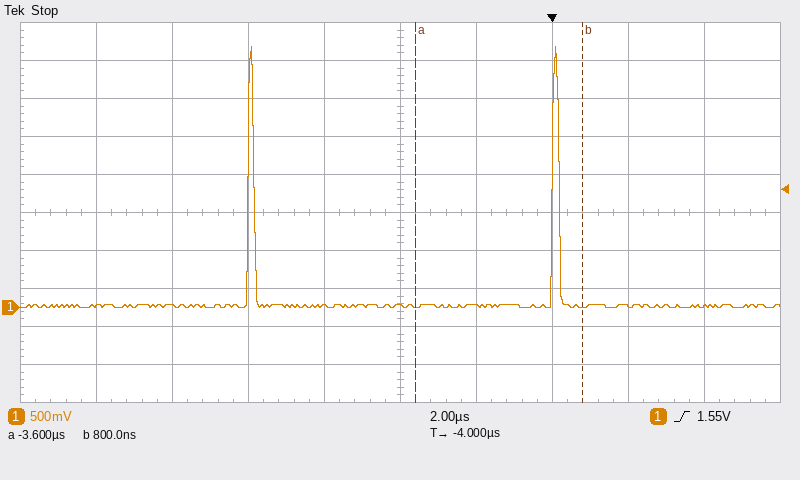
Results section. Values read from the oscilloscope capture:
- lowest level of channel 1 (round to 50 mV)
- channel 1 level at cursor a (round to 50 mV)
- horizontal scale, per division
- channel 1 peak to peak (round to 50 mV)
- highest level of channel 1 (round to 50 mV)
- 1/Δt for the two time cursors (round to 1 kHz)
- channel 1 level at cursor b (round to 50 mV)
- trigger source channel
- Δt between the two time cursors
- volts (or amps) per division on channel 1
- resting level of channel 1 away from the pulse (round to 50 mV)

0 mV
0 mV
2 µs
3.45 V
3.45 V
227 kHz
0 mV
channel 1
4.4 µs
500 mV
0 mV
